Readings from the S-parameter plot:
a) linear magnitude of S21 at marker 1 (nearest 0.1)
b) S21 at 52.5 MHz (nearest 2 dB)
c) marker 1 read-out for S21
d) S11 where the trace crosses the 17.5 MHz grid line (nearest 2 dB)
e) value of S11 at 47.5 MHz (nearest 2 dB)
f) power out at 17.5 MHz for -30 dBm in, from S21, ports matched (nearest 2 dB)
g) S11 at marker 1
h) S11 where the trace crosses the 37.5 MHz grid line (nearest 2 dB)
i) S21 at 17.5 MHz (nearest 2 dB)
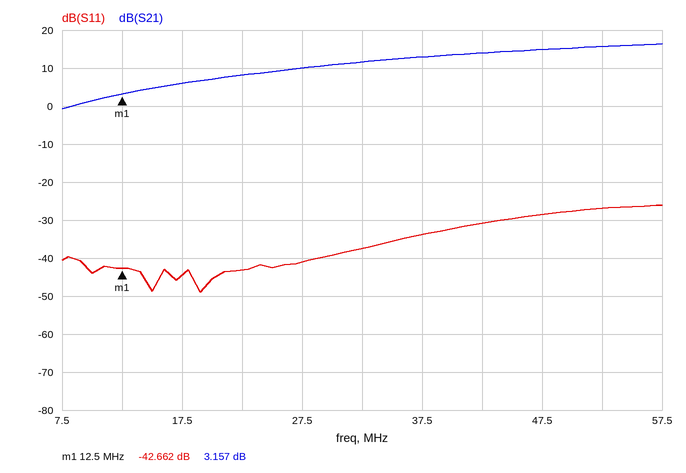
1.4
16 dB
3.157 dB
-44 dB
-28 dB
-24 dBm
-42.662 dB
-34 dB
6 dB
